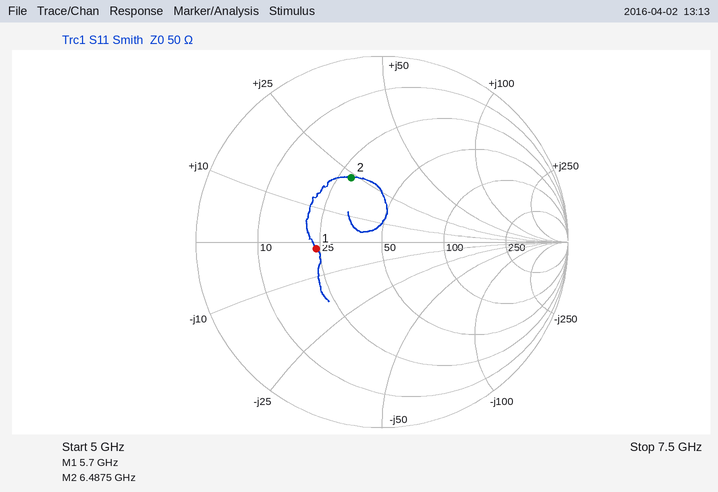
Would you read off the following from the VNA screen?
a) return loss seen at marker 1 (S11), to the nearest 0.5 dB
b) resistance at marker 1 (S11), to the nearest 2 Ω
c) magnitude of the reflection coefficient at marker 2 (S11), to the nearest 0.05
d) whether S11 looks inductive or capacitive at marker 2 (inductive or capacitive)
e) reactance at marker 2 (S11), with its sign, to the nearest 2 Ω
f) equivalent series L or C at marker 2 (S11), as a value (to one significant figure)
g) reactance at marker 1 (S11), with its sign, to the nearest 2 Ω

9.0 dB
24 Ω
0.40
inductive
+24 Ω
600 pH
-2 Ω
